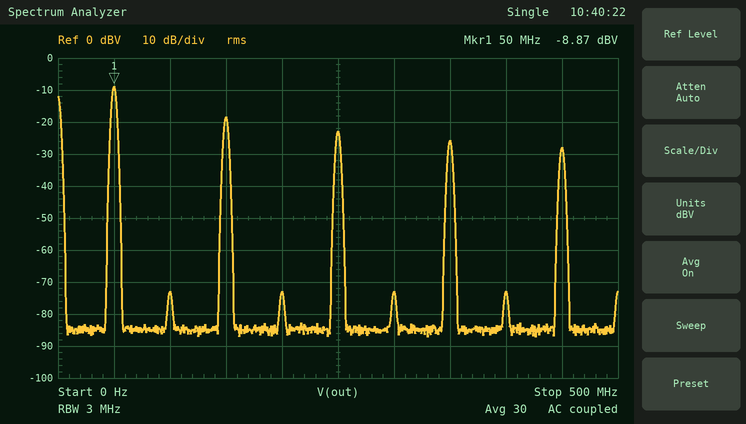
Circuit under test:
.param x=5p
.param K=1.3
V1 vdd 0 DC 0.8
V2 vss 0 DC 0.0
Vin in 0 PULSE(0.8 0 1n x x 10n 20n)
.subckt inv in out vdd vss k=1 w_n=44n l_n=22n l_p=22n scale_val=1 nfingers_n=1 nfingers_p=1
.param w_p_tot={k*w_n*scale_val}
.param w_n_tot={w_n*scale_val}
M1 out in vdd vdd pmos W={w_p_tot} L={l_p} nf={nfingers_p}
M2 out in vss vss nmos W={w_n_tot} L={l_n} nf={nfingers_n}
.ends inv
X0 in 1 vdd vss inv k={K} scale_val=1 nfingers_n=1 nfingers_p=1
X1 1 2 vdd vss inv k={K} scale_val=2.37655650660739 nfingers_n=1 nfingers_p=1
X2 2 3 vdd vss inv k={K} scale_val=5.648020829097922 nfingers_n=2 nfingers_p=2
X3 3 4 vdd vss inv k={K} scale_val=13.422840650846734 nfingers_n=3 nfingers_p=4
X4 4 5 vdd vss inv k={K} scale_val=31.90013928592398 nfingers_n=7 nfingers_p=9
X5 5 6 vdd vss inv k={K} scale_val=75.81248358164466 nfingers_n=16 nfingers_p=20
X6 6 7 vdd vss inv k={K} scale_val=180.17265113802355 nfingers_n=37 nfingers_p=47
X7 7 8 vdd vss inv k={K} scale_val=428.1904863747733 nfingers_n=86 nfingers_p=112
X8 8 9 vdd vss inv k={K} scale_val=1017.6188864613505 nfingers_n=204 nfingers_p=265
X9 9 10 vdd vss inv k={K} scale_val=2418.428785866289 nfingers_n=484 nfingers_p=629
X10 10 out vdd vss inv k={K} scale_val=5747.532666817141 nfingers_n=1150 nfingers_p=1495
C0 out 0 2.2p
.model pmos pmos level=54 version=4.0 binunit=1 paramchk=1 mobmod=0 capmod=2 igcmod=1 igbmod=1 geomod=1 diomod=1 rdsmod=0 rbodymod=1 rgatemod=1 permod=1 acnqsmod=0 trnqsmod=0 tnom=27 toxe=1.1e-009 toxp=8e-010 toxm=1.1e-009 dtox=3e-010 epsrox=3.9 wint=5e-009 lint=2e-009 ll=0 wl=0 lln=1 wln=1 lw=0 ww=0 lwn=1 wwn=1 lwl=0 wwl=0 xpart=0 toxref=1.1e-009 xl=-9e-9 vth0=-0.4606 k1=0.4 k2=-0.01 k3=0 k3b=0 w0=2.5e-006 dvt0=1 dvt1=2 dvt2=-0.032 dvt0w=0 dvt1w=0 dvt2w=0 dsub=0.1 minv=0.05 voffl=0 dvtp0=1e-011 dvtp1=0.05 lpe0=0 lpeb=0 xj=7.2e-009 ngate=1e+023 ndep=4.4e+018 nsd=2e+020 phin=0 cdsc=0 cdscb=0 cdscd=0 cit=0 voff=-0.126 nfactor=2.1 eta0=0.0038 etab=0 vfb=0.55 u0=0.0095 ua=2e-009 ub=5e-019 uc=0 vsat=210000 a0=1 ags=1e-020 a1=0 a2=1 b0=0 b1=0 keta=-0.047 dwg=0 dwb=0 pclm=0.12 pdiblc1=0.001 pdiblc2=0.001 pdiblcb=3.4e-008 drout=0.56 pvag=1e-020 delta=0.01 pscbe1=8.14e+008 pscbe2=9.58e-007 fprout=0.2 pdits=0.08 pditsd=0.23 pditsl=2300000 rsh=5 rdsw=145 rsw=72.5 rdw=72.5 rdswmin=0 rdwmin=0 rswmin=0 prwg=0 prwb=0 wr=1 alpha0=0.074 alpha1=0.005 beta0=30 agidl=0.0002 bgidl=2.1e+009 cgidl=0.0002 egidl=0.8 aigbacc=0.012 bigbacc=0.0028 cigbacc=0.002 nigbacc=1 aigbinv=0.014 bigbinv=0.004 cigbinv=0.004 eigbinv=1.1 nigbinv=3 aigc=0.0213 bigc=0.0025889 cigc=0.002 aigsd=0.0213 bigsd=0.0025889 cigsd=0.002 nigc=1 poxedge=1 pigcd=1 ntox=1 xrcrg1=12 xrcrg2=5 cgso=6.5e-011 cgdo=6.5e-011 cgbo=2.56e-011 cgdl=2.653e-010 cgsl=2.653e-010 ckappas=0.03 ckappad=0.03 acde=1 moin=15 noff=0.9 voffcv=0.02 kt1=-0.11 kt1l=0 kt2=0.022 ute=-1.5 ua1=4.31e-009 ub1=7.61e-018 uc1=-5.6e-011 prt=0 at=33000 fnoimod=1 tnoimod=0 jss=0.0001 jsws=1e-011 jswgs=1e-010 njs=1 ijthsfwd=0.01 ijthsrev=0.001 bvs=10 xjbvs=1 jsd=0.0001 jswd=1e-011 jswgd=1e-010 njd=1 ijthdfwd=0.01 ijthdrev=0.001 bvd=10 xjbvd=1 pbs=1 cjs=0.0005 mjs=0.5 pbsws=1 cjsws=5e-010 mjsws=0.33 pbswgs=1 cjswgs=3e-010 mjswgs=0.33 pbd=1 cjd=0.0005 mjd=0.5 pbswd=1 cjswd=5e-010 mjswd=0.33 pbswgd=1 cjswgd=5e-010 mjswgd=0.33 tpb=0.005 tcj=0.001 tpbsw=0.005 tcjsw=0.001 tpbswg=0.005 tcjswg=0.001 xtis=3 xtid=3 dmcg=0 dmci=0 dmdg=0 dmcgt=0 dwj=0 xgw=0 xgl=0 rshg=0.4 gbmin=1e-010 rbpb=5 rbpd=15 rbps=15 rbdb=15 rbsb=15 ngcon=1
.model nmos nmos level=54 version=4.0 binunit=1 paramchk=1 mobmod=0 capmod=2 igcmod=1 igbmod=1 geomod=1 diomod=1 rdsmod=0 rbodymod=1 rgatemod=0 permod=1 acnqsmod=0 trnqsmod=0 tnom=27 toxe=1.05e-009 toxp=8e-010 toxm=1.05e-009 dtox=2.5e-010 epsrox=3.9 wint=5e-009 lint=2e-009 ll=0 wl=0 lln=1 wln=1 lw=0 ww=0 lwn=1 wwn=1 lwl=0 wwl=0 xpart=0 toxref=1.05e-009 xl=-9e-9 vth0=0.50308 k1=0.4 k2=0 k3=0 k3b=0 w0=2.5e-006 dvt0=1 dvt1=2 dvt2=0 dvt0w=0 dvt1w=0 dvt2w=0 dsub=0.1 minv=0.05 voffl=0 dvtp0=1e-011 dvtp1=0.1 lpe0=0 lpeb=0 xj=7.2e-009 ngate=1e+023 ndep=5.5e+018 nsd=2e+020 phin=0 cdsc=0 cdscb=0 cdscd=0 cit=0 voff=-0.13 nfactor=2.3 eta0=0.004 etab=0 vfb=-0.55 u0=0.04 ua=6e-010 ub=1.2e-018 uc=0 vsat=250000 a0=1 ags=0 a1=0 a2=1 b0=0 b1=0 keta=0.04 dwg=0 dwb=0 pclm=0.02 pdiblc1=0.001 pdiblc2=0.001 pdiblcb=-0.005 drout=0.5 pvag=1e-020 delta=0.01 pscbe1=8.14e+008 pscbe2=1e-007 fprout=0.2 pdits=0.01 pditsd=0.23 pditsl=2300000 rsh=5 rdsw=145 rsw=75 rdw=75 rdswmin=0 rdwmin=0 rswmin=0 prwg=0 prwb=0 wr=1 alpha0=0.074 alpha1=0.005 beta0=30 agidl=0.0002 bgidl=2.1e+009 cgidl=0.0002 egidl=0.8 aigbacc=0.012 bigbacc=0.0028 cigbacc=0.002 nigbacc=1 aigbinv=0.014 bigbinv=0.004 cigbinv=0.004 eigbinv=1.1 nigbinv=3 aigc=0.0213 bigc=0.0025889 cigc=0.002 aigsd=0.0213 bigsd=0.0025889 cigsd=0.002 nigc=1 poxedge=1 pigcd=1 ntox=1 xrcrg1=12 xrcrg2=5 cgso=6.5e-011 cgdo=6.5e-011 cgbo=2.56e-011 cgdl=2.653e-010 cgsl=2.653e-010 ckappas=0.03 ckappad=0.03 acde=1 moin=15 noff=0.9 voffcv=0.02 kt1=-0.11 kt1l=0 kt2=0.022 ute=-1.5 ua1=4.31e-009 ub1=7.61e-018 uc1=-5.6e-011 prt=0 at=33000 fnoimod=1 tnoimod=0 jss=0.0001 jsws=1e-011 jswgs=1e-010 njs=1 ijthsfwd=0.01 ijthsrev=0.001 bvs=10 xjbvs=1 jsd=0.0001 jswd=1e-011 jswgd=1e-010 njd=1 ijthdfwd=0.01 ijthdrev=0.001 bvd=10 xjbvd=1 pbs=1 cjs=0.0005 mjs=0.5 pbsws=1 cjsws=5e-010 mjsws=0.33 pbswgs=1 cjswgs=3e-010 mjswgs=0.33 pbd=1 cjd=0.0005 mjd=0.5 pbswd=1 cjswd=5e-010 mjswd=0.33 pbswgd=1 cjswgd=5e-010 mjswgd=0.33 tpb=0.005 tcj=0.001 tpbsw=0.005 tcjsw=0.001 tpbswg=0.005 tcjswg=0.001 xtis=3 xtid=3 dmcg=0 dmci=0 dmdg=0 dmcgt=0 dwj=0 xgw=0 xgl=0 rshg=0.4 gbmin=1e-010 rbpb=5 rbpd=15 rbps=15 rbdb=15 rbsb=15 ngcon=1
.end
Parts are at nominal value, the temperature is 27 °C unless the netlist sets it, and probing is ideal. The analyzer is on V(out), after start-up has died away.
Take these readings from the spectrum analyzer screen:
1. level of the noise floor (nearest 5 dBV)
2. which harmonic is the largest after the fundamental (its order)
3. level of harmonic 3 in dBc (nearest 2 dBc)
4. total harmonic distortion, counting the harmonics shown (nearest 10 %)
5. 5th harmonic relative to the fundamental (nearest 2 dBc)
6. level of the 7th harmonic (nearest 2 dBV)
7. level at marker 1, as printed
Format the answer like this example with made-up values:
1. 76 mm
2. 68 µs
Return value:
1. -85 dBV
2. 3
3. -10 dBc
4. 40 %
5. -14 dBc
6. -26 dBV
7. -8.87 dBV
